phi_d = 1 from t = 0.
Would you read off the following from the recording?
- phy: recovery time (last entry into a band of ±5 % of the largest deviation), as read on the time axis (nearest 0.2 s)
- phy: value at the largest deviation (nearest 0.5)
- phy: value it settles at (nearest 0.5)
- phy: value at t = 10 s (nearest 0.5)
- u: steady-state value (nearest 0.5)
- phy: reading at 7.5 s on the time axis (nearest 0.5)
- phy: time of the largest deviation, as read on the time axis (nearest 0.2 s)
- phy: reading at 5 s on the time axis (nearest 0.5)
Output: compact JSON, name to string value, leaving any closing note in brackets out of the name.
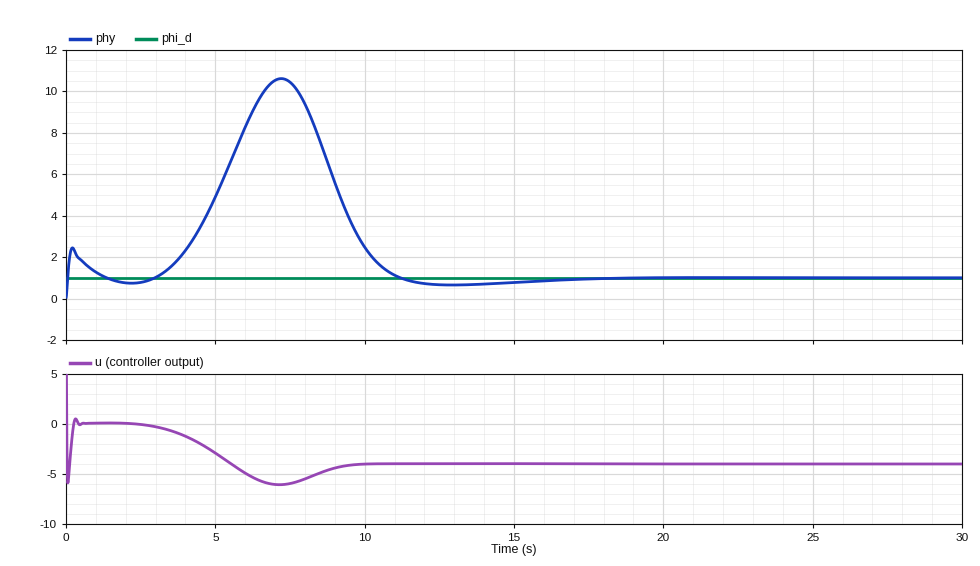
{"phy: recovery time (last entry into a band of ±5 % of the largest deviation), as read on the time axis": "10.6 s", "phy: value at the largest deviation": "10.5", "phy: value it settles at": "1.0", "phy: value at t = 10 s": "2.5", "u: steady-state value": "-4.0", "phy: reading at 7.5 s on the time axis": "10.5", "phy: time of the largest deviation, as read on the time axis": "7.2 s", "phy: reading at 5 s on the time axis": "5.0"}
